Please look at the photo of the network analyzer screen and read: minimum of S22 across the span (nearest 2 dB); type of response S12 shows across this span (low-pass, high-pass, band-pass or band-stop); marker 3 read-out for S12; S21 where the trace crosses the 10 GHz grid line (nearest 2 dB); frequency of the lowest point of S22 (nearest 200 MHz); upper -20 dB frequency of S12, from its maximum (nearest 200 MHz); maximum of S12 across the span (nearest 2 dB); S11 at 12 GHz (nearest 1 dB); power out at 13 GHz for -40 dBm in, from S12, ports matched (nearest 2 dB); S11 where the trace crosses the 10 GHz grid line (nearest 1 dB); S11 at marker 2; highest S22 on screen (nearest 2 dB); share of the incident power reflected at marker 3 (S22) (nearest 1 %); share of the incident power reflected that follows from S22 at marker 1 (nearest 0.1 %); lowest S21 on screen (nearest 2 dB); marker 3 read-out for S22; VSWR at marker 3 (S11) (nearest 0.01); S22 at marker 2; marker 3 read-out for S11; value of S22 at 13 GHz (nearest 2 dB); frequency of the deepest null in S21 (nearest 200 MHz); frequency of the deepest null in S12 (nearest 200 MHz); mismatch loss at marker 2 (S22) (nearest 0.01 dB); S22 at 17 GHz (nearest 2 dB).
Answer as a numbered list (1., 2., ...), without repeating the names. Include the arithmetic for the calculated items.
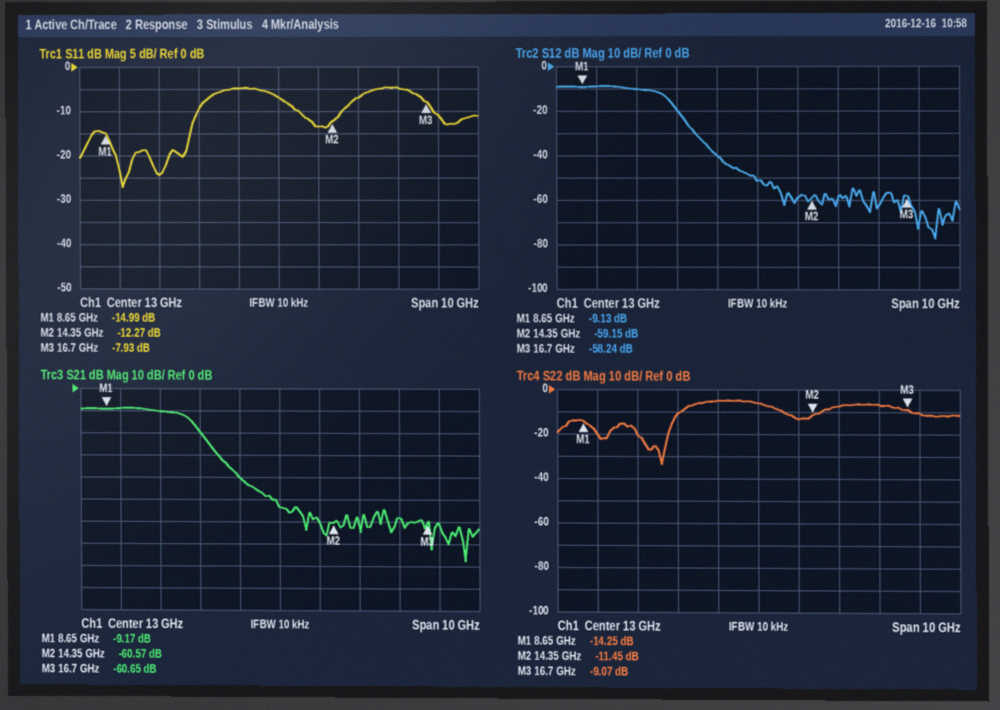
1. -34 dB
2. low-pass
3. -58.24 dB
4. -10 dB
5. 10.6 GHz
6. 11.4 GHz
7. -8 dB
8. -5 dB
9. -40 dBm + (-52 dB) = -92 dBm
10. -24 dB
11. -12.27 dB
12. -4 dB
13. 10^(-9.07/10) ≈ 12 %
14. 10^(-14.25/10) ≈ 3.8 %
15. -78 dB
16. -9.07 dB
17. (1 + 0.4013)/(1 − 0.4013) ≈ 2.34
18. -11.45 dB
19. -7.93 dB
20. -6 dB
21. 17.6 GHz
22. 17.4 GHz
23. −10 log10(1 − 10^(-11.45/10)) ≈ 0.32 dB
24. -10 dB
